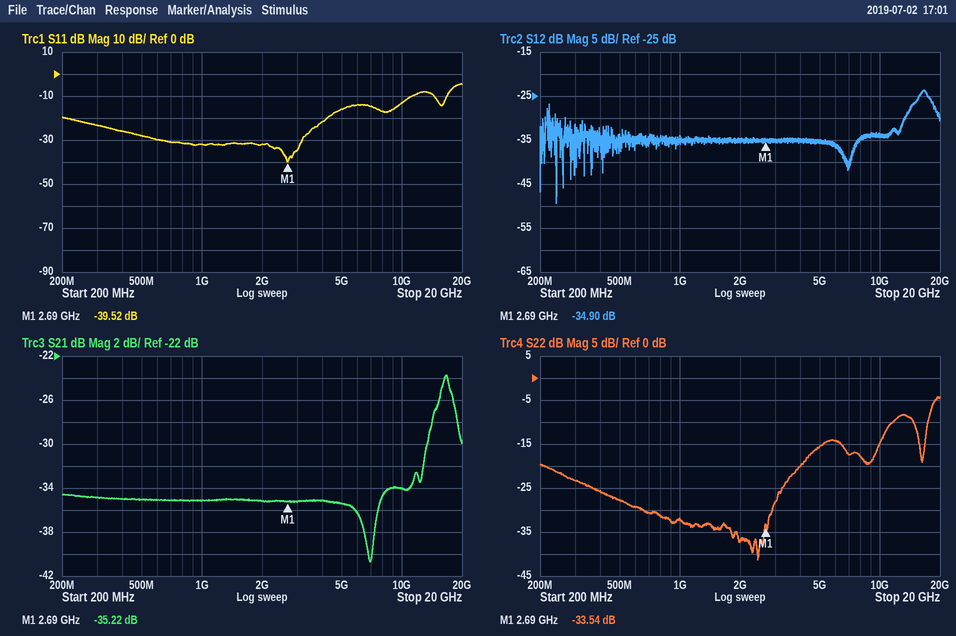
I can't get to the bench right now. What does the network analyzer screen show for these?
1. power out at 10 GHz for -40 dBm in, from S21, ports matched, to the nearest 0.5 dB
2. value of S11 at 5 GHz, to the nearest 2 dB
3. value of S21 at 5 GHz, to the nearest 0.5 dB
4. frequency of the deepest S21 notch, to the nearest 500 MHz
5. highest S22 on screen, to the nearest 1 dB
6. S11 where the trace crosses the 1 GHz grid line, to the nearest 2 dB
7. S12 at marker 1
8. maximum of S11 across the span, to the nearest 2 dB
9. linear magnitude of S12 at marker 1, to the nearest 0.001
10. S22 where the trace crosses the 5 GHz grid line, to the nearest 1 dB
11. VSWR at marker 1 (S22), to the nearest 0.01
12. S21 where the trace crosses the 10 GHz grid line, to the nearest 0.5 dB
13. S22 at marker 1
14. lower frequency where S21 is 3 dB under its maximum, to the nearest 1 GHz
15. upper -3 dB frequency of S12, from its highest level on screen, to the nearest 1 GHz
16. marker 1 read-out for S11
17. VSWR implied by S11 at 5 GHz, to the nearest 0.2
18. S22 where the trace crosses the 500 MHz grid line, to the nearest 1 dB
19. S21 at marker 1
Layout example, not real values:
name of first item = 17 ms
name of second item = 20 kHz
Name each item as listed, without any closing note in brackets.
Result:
power out at 10 GHz for -40 dBm in, from S21, ports matched, to the nearest 0.5 dB = -74.0 dBm
value of S11 at 5 GHz, to the nearest 2 dB = -16 dB
value of S21 at 5 GHz, to the nearest 0.5 dB = -35.5 dB
frequency of the deepest S21 notch, to the nearest 500 MHz = 7.0 GHz
highest S22 on screen, to the nearest 1 dB = -4 dB
S11 where the trace crosses the 1 GHz grid line, to the nearest 2 dB = -32 dB
S12 at marker 1 = -34.90 dB
maximum of S11 across the span, to the nearest 2 dB = -4 dB
linear magnitude of S12 at marker 1, to the nearest 0.001 = 0.018
S22 where the trace crosses the 5 GHz grid line, to the nearest 1 dB = -16 dB
VSWR at marker 1 (S22), to the nearest 0.01 = 1.04
S21 where the trace crosses the 10 GHz grid line, to the nearest 0.5 dB = -34.0 dB
S22 at marker 1 = -33.54 dB
lower frequency where S21 is 3 dB under its maximum, to the nearest 1 GHz = 15 GHz
upper -3 dB frequency of S12, from its highest level on screen, to the nearest 1 GHz = 18 GHz
marker 1 read-out for S11 = -39.52 dB
VSWR implied by S11 at 5 GHz, to the nearest 0.2 = 1.4
S22 where the trace crosses the 500 MHz grid line, to the nearest 1 dB = -28 dB
S21 at marker 1 = -35.22 dB
